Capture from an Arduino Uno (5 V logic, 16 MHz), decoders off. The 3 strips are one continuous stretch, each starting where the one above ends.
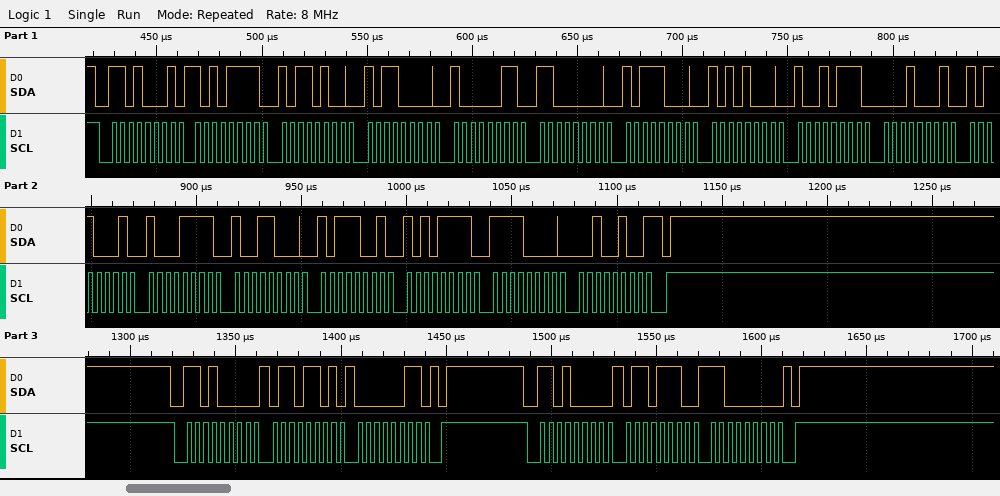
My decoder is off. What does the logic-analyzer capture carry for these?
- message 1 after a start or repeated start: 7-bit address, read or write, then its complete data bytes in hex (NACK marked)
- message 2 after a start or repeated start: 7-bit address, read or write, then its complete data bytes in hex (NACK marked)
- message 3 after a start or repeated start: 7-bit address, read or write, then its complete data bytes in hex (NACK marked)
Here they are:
0x68 read: AF B4 B0 83 C0 B8 A8 97 11 B1 8F 98 B9 AF F0 24 NACK
0x68 write: 6D 03
0x68 write: 6E C0
